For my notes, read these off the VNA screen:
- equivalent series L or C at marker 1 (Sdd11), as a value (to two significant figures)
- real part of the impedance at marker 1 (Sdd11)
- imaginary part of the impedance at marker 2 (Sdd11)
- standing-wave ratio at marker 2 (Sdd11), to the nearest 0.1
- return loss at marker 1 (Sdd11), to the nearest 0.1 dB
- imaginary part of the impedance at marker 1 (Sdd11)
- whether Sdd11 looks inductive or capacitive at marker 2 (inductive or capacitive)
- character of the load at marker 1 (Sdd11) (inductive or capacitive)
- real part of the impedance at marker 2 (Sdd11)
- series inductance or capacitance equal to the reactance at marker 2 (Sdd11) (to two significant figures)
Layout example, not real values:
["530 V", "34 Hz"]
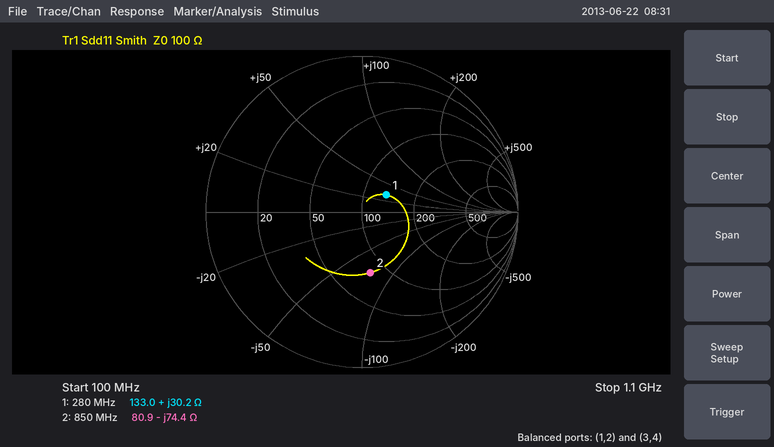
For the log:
["17 nH", "133.0 Ω", "-74.4 Ω", "2.3", "14.4 dB", "+30.2 Ω", "capacitive", "inductive", "80.9 Ω", "2.5 pF"]
